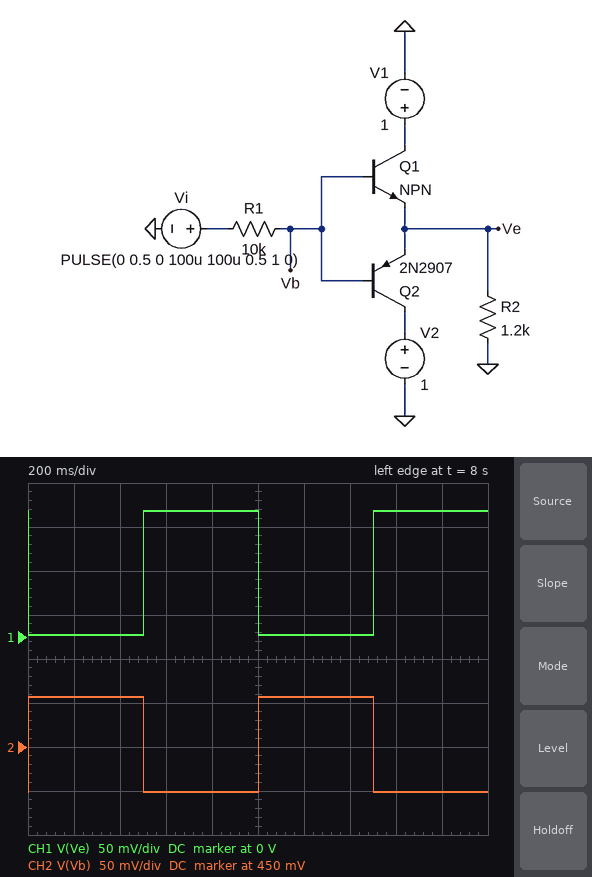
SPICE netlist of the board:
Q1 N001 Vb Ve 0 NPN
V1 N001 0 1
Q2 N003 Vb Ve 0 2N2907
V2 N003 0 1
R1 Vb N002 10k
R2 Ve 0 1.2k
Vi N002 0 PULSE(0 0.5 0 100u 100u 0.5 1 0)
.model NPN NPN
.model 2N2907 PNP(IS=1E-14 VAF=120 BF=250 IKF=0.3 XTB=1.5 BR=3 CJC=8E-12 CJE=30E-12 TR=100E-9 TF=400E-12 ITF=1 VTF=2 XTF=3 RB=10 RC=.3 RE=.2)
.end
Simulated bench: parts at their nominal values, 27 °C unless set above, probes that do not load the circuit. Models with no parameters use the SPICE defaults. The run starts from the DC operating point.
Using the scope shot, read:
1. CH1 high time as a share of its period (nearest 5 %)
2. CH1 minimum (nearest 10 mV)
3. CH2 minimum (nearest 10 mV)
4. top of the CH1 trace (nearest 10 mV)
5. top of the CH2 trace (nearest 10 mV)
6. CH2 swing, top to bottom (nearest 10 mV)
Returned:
50 %
0 V
400 mV
140 mV
510 mV
110 mV
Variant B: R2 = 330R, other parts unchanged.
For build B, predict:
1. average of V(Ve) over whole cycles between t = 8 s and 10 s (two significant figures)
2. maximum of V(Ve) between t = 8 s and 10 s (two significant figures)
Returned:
20 mV
39 mV
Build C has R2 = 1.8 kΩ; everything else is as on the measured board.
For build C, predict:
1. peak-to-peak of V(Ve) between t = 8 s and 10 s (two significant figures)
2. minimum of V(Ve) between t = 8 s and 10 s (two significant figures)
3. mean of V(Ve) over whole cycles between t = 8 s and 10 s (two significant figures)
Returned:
210 mV
3.5 mV
110 mV
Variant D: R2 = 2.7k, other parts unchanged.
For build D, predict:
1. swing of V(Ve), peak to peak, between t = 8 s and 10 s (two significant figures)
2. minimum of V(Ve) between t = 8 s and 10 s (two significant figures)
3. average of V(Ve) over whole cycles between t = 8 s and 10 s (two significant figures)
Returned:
320 mV
5.2 mV
160 mV
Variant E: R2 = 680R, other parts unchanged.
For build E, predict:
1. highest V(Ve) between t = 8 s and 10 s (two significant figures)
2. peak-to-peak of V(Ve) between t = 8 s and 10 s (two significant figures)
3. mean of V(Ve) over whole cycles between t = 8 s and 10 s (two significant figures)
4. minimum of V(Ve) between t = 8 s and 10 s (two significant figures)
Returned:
81 mV
80 mV
41 mV
1.3 mV
